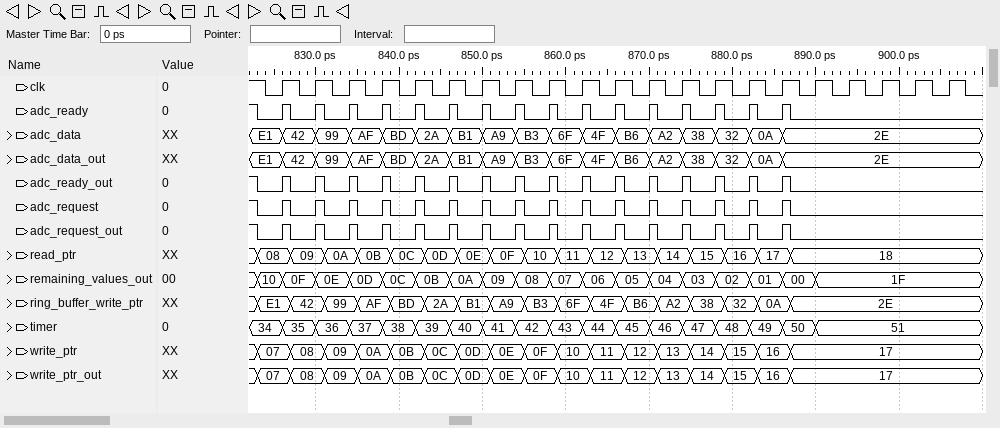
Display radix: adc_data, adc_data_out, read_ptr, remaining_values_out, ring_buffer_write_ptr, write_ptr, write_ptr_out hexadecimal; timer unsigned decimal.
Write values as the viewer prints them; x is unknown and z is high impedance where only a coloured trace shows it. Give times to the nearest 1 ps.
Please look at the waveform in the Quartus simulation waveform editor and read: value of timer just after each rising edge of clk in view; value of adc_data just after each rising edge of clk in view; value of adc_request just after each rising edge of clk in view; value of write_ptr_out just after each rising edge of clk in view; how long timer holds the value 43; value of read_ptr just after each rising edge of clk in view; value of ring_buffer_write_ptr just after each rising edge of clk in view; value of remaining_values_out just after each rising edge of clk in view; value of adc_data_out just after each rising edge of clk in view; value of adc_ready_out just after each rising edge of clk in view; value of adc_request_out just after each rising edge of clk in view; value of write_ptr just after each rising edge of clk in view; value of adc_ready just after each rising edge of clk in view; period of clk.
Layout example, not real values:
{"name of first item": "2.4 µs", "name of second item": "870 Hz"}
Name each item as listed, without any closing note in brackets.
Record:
{"value of timer just after each rising edge of clk in view": "35, 36, 37, 38, 39, 40, 41, 42, 43, 44, 45, 46, 47, 48, 49, 50, 51, 51, 51, 51, 51", "value of adc_data just after each rising edge of clk in view": "42, 99, AF, BD, 2A, B1, A9, B3, 6F, 4F, B6, A2, 38, 32, 0A, 2E, 2E, 2E, 2E, 2E, 2E", "value of adc_request just after each rising edge of clk in view": "1 1 1 1 1 1 1 1 1 1 1 1 1 1 1 1 0 0 0 0 0", "value of write_ptr_out just after each rising edge of clk in view": "07, 08, 09, 0A, 0B, 0C, 0D, 0E, 0F, 10, 11, 12, 13, 14, 15, 16, 17, 17, 17, 17, 17", "how long timer holds the value 43": "4 ps", "value of read_ptr just after each rising edge of clk in view": "08, 09, 0A, 0B, 0C, 0D, 0E, 0F, 10, 11, 12, 13, 14, 15, 16, 17, 18, 18, 18, 18, 18", "value of ring_buffer_write_ptr just after each rising edge of clk in view": "E1, 42, 99, AF, BD, 2A, B1, A9, B3, 6F, 4F, B6, A2, 38, 32, 0A, 2E, 2E, 2E, 2E, 2E", "value of remaining_values_out just after each rising edge of clk in view": "0F, 0E, 0D, 0C, 0B, 0A, 09, 08, 07, 06, 05, 04, 03, 02, 01, 00, 1F, 1F, 1F, 1F, 1F", "value of adc_data_out just after each rising edge of clk in view": "42, 99, AF, BD, 2A, B1, A9, B3, 6F, 4F, B6, A2, 38, 32, 0A, 2E, 2E, 2E, 2E, 2E, 2E", "value of adc_ready_out just after each rising edge of clk in view": "1 1 1 1 1 1 1 1 1 1 1 1 1 1 1 1 0 0 0 0 0", "value of adc_request_out just after each rising edge of clk in view": "1 1 1 1 1 1 1 1 1 1 1 1 1 1 1 1 0 0 0 0 0", "value of write_ptr just after each rising edge of clk in view": "07, 08, 09, 0A, 0B, 0C, 0D, 0E, 0F, 10, 11, 12, 13, 14, 15, 16, 17, 17, 17, 17, 17", "value of adc_ready just after each rising edge of clk in view": "1 1 1 1 1 1 1 1 1 1 1 1 1 1 1 1 0 0 0 0 0", "period of clk": "4 ps"}
